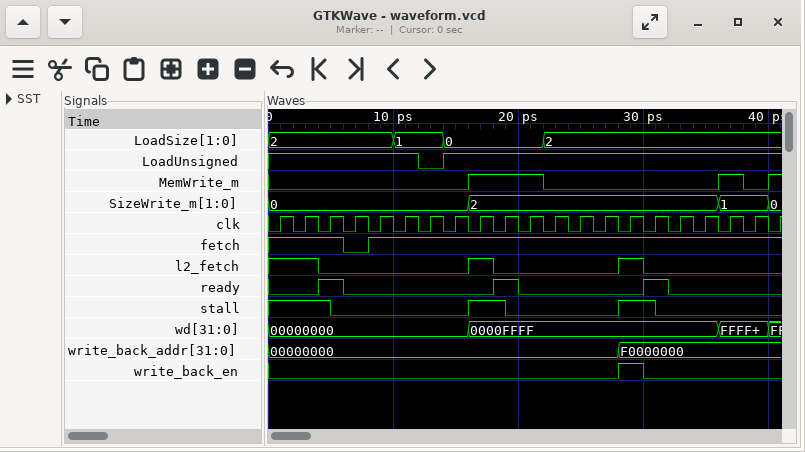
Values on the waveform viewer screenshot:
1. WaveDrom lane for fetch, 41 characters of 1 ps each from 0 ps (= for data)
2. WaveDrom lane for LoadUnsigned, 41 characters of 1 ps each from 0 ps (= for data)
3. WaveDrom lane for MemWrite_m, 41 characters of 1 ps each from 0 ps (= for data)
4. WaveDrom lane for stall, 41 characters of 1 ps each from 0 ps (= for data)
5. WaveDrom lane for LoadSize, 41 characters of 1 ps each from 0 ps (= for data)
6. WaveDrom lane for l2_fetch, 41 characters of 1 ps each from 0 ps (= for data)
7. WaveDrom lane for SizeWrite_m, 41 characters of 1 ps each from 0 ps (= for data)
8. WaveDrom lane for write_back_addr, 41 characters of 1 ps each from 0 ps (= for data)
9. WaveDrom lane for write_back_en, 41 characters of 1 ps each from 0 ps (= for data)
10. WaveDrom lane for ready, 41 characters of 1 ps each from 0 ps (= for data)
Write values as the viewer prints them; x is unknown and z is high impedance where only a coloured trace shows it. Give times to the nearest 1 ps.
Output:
{name: 'fetch', wave: '1.....0.1................................'}
{name: 'LoadUnsigned', wave: '1...........0.1..........................'}
{name: 'MemWrite_m', wave: '0...............1.....0.............1.0.1'}
{name: 'stall', wave: '1....0..........1..0........1..0.........'}
{name: 'LoadSize', wave: '=.........=...=.......=..................', data: '2 1 0 2'}
{name: 'l2_fetch', wave: '1...0...........1.0.........1.0..........'}
{name: 'SizeWrite_m', wave: '=...............=...................=...=', data: '0 2 1 0'}
{name: 'write_back_addr', wave: '=...........................=............', data: '00000000 F0000000'}
{name: 'write_back_en', wave: '0...........................1.0..........'}
{name: 'ready', wave: '0...1.0...........1.0.........1.0........'}
